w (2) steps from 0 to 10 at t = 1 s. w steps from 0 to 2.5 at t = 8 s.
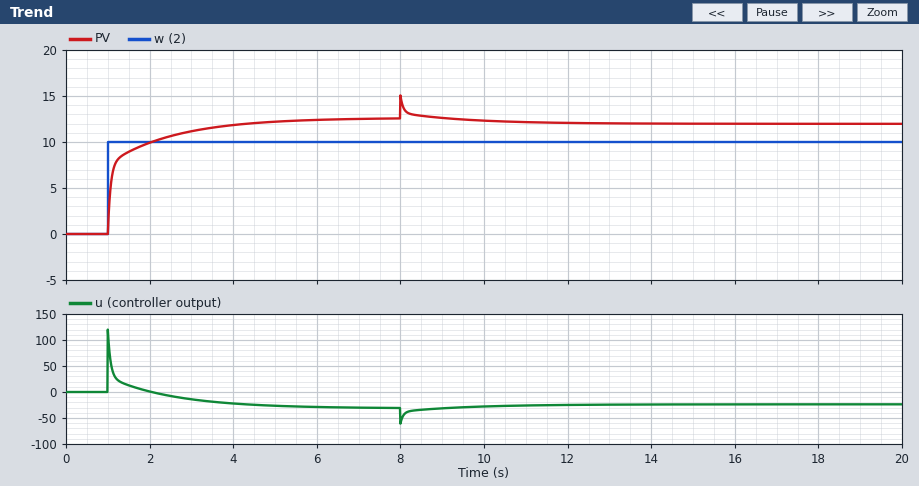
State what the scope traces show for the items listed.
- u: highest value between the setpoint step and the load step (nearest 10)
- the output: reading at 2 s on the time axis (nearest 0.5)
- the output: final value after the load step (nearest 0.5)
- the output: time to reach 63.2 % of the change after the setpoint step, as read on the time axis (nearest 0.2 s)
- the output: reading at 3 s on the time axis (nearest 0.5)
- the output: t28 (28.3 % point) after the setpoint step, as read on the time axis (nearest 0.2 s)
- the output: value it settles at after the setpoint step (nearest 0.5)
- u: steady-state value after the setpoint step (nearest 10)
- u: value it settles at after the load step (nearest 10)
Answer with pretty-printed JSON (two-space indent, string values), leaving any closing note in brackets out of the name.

{
  "u: highest value between the setpoint step and the load step": "120",
  "the output: reading at 2 s on the time axis": "10.0",
  "the output: final value after the load step": "12.0",
  "the output: time to reach 63.2 % of the change after the setpoint step, as read on the time axis": "1.2 s",
  "the output: reading at 3 s on the time axis": "11.0",
  "the output: t28 (28.3 % point) after the setpoint step, as read on the time axis": "1.0 s",
  "the output: value it settles at after the setpoint step": "12.5",
  "u: steady-state value after the setpoint step": "-30",
  "u: value it settles at after the load step": "-20"
}
